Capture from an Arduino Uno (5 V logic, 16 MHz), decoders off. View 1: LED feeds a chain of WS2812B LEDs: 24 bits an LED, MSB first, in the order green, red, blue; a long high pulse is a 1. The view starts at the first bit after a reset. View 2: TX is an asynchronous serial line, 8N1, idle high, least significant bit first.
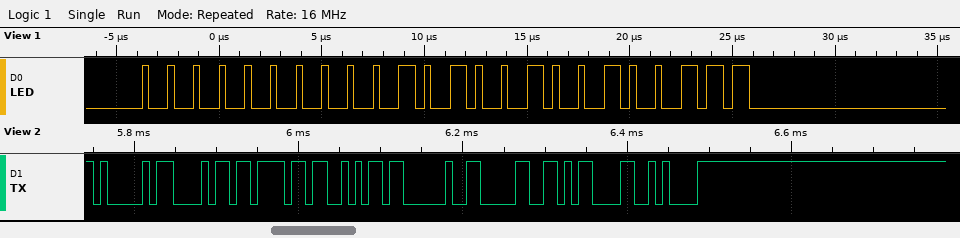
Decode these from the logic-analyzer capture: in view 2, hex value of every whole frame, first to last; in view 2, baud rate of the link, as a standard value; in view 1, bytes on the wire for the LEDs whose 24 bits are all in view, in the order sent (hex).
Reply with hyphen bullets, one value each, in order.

- 41 68 6F 6A 20 30 0D 0A
- 115200 baud
- 00 29 27
